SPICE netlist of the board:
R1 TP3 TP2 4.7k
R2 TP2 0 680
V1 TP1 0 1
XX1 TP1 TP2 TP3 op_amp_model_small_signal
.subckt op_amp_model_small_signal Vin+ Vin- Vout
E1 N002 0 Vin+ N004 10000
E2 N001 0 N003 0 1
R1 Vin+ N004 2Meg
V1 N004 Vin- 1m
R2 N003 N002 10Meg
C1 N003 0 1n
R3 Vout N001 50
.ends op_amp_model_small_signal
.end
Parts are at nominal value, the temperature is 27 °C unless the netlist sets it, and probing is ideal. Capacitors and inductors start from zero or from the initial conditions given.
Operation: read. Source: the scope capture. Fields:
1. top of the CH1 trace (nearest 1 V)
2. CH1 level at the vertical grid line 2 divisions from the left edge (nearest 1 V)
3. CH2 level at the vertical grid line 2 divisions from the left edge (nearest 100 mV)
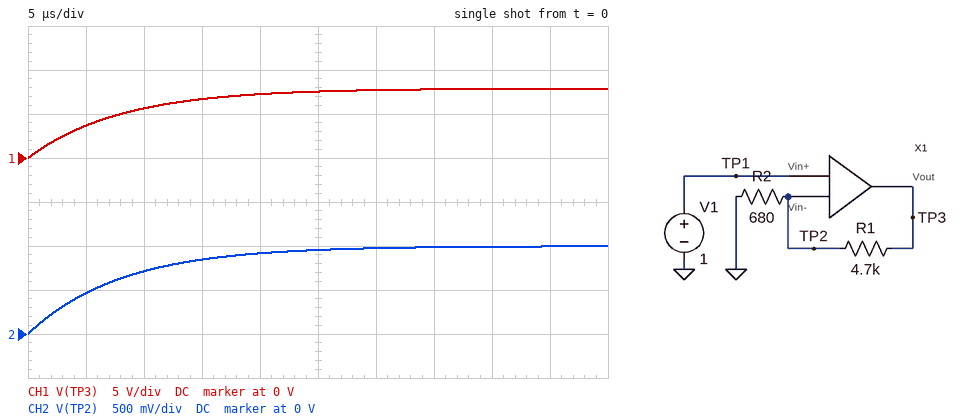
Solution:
8 V
6 V
700 mV
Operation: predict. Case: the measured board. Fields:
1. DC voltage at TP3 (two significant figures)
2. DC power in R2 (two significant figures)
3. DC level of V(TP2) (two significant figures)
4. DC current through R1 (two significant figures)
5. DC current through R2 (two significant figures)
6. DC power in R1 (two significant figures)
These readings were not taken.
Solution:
7.9 V
1.5 mW
1.0 V
1.5 mA
1.5 mA
10 mW
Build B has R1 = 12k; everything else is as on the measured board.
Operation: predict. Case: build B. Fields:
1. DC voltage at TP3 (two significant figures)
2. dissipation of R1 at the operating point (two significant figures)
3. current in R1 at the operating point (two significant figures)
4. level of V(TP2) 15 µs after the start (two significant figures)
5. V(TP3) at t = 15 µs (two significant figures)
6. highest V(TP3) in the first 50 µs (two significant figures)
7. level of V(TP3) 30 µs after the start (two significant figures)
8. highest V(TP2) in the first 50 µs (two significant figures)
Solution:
19 V
26 mW
1.5 mA
550 mV
10 V
17 V
15 V
930 mV
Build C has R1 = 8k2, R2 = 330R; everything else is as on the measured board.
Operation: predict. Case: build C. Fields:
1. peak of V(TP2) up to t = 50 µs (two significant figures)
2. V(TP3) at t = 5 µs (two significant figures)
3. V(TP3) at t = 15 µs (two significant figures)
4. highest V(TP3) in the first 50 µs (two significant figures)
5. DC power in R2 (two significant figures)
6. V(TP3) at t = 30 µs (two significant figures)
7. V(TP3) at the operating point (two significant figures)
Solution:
850 mV
4.5 V
11 V
22 V
3.0 mW
18 V
26 V
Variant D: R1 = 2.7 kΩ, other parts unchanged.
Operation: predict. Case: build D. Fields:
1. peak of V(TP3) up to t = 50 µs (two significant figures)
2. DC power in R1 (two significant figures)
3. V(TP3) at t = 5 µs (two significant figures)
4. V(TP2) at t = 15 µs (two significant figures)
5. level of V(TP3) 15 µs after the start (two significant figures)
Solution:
5.0 V
5.8 mW
3.1 V
950 mV
4.7 V
